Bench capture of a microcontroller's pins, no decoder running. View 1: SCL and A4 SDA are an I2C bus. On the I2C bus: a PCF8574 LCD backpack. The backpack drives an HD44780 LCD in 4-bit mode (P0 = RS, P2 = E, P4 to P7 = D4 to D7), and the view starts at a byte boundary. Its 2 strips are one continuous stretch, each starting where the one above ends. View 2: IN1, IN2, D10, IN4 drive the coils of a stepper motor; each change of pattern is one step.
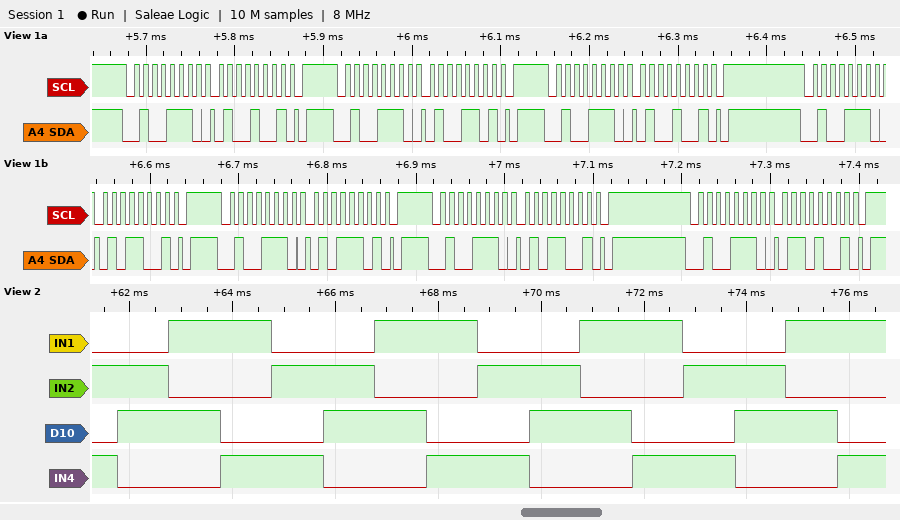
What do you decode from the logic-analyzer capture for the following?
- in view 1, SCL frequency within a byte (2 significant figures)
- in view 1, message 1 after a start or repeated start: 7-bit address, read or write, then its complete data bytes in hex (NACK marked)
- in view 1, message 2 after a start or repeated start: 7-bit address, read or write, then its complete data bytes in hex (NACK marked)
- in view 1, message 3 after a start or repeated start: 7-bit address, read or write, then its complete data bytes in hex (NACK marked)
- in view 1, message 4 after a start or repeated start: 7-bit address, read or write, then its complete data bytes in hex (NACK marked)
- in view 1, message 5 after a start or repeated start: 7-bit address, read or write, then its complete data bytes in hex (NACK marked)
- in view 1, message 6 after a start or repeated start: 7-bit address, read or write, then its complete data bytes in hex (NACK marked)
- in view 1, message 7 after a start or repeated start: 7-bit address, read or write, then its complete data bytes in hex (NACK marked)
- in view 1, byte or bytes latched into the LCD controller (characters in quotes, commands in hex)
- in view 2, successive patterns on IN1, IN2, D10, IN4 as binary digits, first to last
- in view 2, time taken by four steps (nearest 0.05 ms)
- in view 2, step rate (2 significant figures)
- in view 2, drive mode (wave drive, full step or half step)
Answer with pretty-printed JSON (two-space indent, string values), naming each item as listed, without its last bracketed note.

{
  "in view 1, SCL frequency within a byte": "100 kHz",
  "in view 1, message 1 after a start or repeated start: 7-bit address, read or write, then its complete data bytes in hex": "0x27 write: 49",
  "in view 1, message 2 after a start or repeated start: 7-bit address, read or write, then its complete data bytes in hex": "0x27 write: 4D",
  "in view 1, message 3 after a start or repeated start: 7-bit address, read or write, then its complete data bytes in hex": "0x27 write: 49",
  "in view 1, message 4 after a start or repeated start: 7-bit address, read or write, then its complete data bytes in hex": "0x27 write: 59",
  "in view 1, message 5 after a start or repeated start: 7-bit address, read or write, then its complete data bytes in hex": "0x27 write: 5D",
  "in view 1, message 6 after a start or repeated start: 7-bit address, read or write, then its complete data bytes in hex": "0x27 write: 59",
  "in view 1, message 7 after a start or repeated start: 7-bit address, read or write, then its complete data bytes in hex": "0x27 write: 69",
  "in view 1, byte or bytes latched into the LCD controller": "'E'",
  "in view 2, successive patterns on IN1, IN2, D10, IN4 as binary digits, first to last": "0101 0110 1010 1001 0101 0110 1010 1001 0101 0110 1010 1001 0101 0110 1010 1001",
  "in view 2, time taken by four steps": "4.00 ms",
  "in view 2, step rate": "1000 steps/s",
  "in view 2, drive mode": "full step"
}
